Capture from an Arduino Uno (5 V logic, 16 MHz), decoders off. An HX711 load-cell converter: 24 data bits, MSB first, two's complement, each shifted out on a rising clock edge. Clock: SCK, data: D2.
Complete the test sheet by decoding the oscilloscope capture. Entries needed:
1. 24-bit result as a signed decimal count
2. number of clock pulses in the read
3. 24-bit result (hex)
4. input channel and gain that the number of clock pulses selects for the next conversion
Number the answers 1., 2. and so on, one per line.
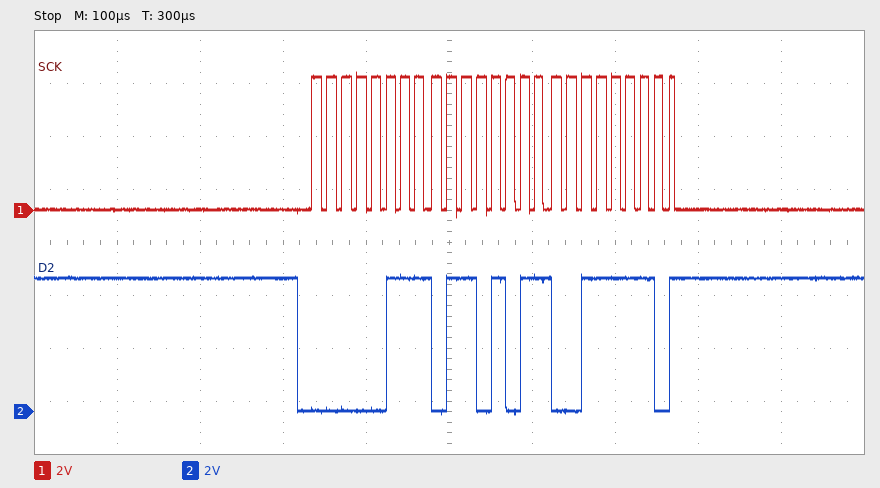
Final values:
1. 486206
2. 25
3. 0x076B3E
4. channel A, gain 128
